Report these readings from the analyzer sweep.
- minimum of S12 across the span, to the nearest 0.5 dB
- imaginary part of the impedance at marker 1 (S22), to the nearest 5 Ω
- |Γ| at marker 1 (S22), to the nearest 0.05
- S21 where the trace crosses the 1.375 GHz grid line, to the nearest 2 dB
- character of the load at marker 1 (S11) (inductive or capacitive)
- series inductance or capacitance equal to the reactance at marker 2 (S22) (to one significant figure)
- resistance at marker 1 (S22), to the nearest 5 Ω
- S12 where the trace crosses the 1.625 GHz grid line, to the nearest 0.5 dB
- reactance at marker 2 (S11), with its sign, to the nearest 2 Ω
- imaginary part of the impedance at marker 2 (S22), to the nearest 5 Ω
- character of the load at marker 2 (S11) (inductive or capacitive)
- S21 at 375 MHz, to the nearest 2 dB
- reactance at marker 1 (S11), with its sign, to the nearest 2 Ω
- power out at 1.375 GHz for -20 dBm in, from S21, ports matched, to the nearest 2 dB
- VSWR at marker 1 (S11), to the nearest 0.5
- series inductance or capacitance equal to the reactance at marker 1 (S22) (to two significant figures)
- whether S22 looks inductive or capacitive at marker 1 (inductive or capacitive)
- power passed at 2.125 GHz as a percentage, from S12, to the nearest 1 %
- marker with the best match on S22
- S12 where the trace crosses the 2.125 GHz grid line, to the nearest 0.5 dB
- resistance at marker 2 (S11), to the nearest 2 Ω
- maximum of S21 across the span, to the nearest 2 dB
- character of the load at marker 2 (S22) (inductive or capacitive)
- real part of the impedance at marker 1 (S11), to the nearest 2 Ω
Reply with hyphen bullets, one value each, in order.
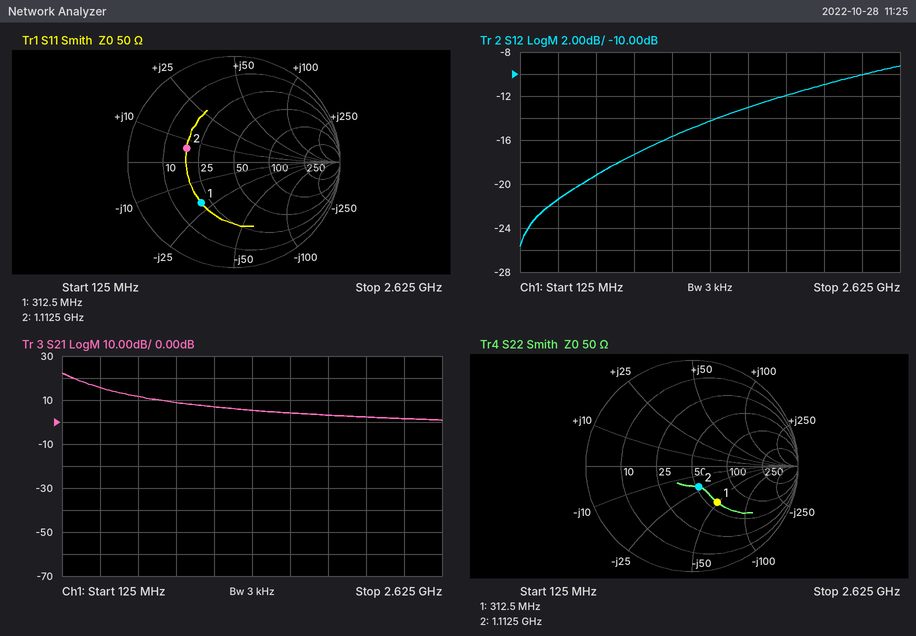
- -25.5 dB
- -50 Ω
- 0.40
- 6 dB
- capacitive
- 7 pF
- 60 Ω
- -13.0 dB
- +6 Ω
- -20 Ω
- inductive
- 16 dB
- -20 Ω
- -14 dBm
- 3.0
- 10 pF
- capacitive
- 8 %
- marker 2
- -11.0 dB
- 18 Ω
- 22 dB
- capacitive
- 20 Ω
